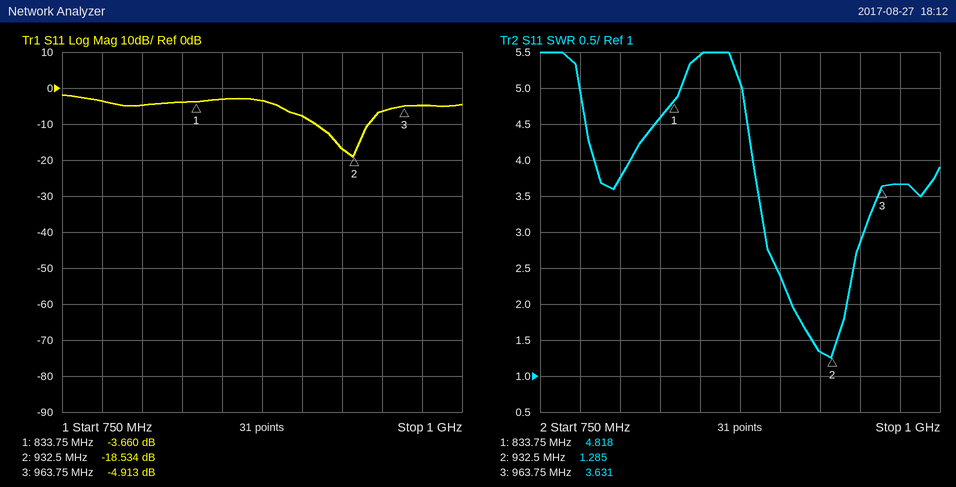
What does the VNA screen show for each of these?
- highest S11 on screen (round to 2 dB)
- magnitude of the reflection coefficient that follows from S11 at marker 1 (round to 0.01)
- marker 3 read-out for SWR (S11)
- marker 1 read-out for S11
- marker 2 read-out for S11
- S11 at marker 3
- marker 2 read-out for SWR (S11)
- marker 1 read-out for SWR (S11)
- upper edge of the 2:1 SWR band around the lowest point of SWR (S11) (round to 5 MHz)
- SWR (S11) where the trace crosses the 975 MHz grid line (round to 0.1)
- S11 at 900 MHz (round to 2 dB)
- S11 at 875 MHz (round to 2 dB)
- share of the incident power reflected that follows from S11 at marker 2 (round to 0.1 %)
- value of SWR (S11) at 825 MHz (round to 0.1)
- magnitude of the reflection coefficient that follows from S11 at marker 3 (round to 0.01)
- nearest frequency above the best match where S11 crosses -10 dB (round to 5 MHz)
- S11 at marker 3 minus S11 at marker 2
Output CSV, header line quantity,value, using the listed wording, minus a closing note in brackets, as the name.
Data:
quantity,value
highest S11 on screen,-2 dB
magnitude of the reflection coefficient that follows from S11 at marker 1,0.66
marker 3 read-out for SWR,3.631
marker 1 read-out for S11,-3.660 dB
marker 2 read-out for S11,-18.534 dB
S11 at marker 3,-4.913 dB
marker 2 read-out for SWR,1.285
marker 1 read-out for SWR,4.818
upper edge of the 2:1 SWR band around the lowest point of SWR (S11),940 MHz
SWR (S11) where the trace crosses the 975 MHz grid line,3.7
S11 at 900 MHz,-8 dB
S11 at 875 MHz,-4 dB
share of the incident power reflected that follows from S11 at marker 2,1.4 %
value of SWR (S11) at 825 MHz,4.6
magnitude of the reflection coefficient that follows from S11 at marker 3,0.57
nearest frequency above the best match where S11 crosses -10 dB,940 MHz
S11 at marker 3 minus S11 at marker 2,13.621 dB
